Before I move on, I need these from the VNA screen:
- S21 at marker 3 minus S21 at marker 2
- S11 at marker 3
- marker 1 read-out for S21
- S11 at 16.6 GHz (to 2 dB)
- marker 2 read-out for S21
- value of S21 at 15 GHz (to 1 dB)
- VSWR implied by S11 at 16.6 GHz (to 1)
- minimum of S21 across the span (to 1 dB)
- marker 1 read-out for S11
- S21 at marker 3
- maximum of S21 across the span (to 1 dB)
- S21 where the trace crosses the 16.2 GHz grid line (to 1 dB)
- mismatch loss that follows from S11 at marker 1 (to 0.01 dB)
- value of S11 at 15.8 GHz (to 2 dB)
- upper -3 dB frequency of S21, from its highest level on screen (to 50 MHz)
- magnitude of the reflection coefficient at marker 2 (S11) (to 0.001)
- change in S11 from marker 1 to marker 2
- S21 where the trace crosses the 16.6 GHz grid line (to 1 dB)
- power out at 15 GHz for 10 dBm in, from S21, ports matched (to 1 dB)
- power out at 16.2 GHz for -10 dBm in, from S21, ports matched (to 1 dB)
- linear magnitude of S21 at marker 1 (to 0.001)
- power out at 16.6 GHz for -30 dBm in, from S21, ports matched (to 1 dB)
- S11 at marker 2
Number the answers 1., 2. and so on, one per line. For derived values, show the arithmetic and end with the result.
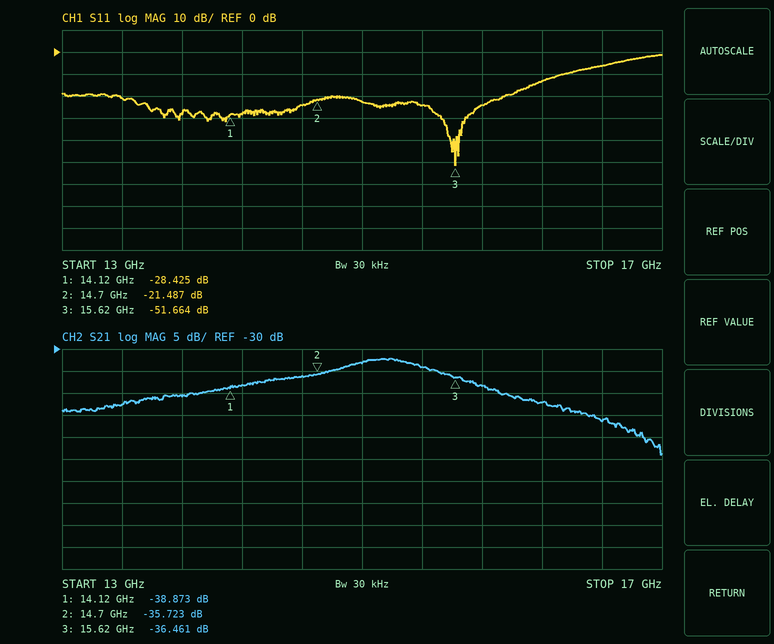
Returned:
1. -36.461 − (-35.723) = -0.738 dB
2. -51.664 dB
3. -38.873 dB
4. -6 dB
5. -35.723 dB
6. -33 dB
7. |Γ| = 10^(-6/20) = 0.5012; VSWR = (1 + 0.5012)/(1 − 0.5012) ≈ 3
8. -54 dB
9. -28.425 dB
10. -36.461 dB
11. -32 dB
12. -42 dB
13. −10 log10(1 − 10^(-28.425/10)) ≈ 0.01 dB
14. -24 dB
15. 15.50 GHz
16. 10^(-21.487/20) ≈ 0.084
17. -21.487 − (-28.425) = 6.938 dB
18. -46 dB
19. 10 dBm + (-33 dB) = -23 dBm
20. -10 dBm + (-42 dB) = -52 dBm
21. 10^(-38.873/20) ≈ 0.011
22. -30 dBm + (-46 dB) = -76 dBm
23. -21.487 dB
